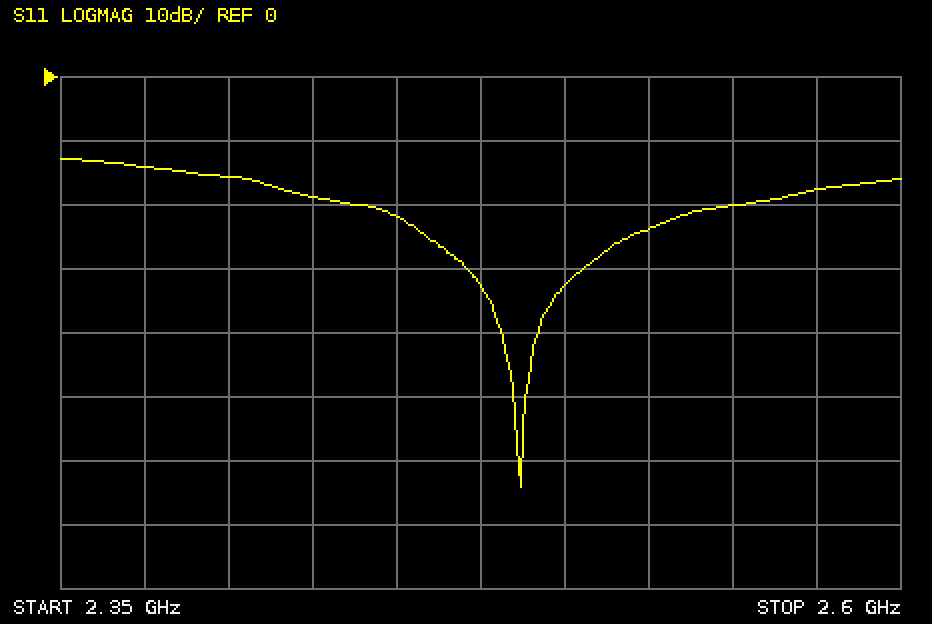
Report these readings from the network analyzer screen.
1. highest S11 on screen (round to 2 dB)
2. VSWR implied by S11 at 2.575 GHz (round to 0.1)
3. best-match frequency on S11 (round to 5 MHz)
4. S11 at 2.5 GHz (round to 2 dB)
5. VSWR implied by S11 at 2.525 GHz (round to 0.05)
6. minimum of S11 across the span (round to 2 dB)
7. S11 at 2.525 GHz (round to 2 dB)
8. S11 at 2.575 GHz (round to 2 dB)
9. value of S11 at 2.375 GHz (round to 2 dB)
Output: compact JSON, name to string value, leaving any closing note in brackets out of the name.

{"highest S11 on screen": "-12 dB", "VSWR implied by S11 at 2.575 GHz": "1.3", "best-match frequency on S11": "2.485 GHz", "S11 at 2.5 GHz": "-32 dB", "VSWR implied by S11 at 2.525 GHz": "1.15", "minimum of S11 across the span": "-64 dB", "S11 at 2.525 GHz": "-24 dB", "S11 at 2.575 GHz": "-18 dB", "value of S11 at 2.375 GHz": "-14 dB"}
